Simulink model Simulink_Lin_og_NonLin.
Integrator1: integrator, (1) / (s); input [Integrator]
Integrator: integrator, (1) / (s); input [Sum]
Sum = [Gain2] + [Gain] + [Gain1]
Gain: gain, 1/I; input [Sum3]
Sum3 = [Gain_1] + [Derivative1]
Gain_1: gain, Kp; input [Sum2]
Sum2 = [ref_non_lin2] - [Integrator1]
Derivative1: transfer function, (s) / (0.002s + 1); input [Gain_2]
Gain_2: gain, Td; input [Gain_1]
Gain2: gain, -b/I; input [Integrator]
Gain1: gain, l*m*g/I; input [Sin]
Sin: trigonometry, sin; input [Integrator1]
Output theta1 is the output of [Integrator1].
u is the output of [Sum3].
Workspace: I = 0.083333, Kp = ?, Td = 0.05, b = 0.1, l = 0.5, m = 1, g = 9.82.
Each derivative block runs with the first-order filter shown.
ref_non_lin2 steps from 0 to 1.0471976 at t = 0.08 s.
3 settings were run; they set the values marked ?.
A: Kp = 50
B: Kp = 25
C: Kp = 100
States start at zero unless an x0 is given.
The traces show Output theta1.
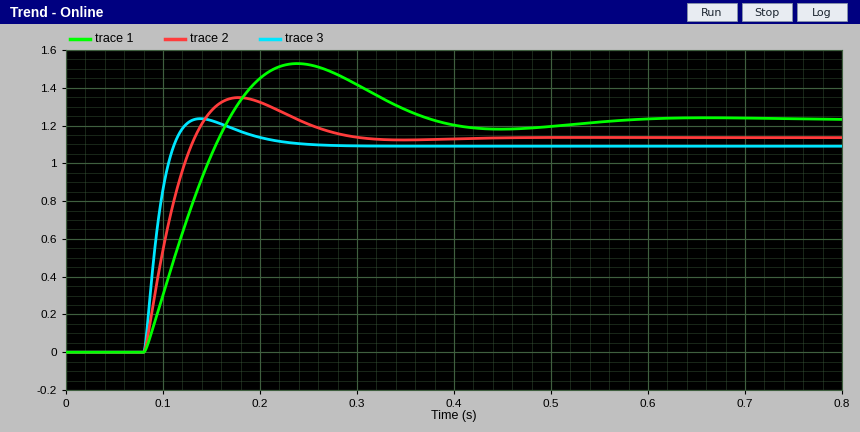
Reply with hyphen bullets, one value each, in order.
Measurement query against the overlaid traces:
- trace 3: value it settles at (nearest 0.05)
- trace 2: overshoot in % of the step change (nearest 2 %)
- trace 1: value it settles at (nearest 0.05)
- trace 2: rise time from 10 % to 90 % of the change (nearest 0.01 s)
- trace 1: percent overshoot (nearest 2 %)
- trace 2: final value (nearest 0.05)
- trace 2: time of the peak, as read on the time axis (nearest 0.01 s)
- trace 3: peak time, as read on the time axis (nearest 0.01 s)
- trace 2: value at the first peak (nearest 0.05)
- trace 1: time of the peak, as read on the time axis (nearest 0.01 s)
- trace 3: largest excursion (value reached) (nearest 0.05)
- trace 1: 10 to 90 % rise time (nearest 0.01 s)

- 1.10
- 18 %
- 1.25
- 0.04 s
- 24 %
- 1.15
- 0.18 s
- 0.14 s
- 1.35
- 0.24 s
- 1.25
- 0.07 s
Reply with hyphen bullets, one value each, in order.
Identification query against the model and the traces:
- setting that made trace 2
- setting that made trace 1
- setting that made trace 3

- A
- B
- C
